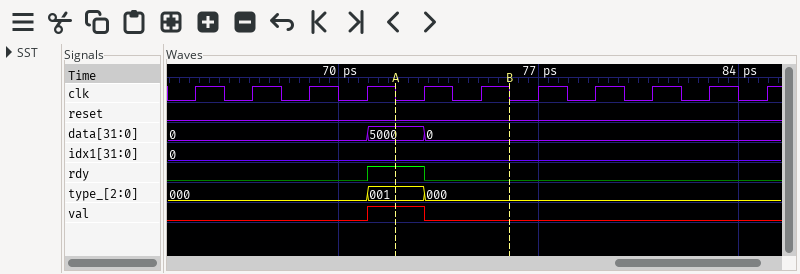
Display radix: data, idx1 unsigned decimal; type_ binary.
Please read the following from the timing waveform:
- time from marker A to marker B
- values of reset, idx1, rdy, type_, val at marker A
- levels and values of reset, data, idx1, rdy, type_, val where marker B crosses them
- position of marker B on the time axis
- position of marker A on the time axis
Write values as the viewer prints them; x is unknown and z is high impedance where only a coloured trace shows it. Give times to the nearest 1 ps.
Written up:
4 ps
reset=0, idx1=0, rdy=1, type_=001, val=1
reset=0, data=0, idx1=0, rdy=0, type_=000, val=0
76 ps
72 ps
